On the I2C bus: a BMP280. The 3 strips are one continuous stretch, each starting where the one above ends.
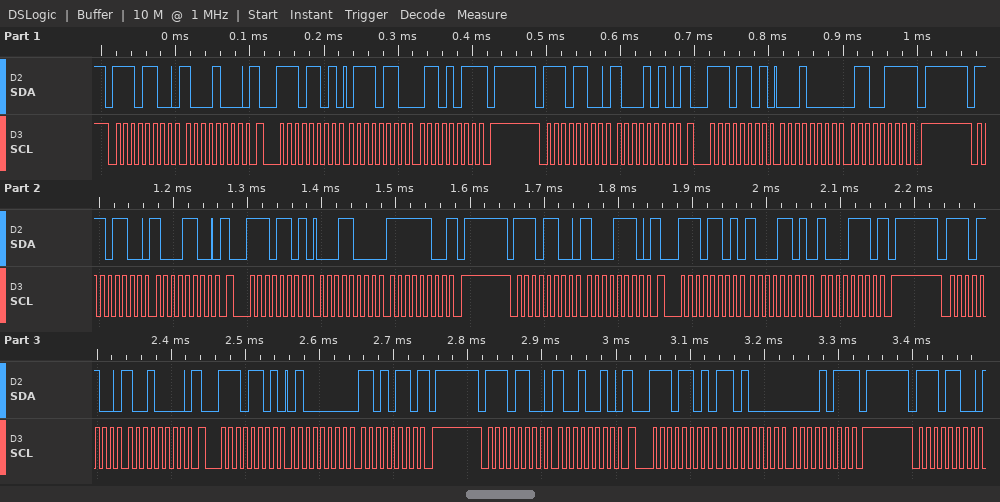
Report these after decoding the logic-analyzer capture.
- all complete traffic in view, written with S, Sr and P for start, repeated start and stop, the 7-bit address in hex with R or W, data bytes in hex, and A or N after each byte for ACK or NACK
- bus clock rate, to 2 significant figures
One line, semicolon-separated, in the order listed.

S 76W A 88 A Sr 76R A 76 A 6B N P S 76W A 8A A Sr 76R A 10 A 67 N P S 76W A 8C A Sr 76R A 18 A FC N P S 76W A 8E A Sr 76R A 8D A 8E N P S 76W A 90 A Sr 76R A 40 A D6 N P S 76W A 92 A Sr 76R A D0 A 0B N P S 76W A; 100 kHz
